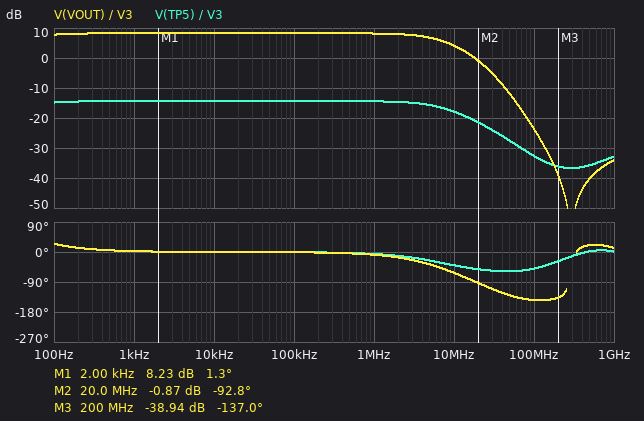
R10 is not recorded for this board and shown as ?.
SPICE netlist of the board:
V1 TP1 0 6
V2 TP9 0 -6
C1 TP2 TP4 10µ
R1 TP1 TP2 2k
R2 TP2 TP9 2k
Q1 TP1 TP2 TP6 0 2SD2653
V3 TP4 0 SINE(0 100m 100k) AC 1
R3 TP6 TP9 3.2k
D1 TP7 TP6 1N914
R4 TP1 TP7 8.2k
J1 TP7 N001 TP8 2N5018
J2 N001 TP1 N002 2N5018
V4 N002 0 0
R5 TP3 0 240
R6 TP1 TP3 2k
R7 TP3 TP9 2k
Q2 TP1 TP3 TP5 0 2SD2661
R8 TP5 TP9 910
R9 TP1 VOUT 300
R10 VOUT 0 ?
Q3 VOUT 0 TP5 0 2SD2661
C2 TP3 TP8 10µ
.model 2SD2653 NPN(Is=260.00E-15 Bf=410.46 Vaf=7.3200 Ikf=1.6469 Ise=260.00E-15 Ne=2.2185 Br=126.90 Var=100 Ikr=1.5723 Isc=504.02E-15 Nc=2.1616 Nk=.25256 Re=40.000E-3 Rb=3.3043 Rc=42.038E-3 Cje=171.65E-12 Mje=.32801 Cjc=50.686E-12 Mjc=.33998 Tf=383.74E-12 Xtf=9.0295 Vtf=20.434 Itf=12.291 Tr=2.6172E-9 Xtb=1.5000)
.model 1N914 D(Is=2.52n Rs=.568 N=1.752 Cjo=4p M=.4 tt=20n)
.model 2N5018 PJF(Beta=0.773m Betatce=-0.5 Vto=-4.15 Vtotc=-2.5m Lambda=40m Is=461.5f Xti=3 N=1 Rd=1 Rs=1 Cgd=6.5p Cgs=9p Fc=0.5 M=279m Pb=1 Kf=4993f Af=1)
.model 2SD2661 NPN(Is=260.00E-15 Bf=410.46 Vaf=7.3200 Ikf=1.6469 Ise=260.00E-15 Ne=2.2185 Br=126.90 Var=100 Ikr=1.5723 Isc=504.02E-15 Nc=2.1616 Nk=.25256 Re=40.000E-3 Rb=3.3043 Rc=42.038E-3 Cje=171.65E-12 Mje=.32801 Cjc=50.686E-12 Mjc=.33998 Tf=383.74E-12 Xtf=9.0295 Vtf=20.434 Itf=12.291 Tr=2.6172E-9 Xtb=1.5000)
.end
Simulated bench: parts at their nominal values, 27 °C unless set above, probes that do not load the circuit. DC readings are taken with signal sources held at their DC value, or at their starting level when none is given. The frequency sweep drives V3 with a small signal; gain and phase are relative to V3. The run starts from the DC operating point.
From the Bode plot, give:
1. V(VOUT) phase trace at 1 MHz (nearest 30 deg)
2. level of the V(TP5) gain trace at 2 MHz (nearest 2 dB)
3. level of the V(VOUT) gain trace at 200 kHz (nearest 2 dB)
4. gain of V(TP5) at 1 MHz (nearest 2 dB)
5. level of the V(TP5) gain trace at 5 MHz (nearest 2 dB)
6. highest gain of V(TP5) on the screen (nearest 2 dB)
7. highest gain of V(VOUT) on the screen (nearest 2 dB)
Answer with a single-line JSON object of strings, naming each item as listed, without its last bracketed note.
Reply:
{"V(VOUT) phase trace at 1 MHz": "0 deg", "level of the V(TP5) gain trace at 2 MHz": "-14 dB", "level of the V(VOUT) gain trace at 200 kHz": "8 dB", "gain of V(TP5) at 1 MHz": "-14 dB", "level of the V(TP5) gain trace at 5 MHz": "-16 dB", "highest gain of V(TP5) on the screen": "-14 dB", "highest gain of V(VOUT) on the screen": "8 dB"}
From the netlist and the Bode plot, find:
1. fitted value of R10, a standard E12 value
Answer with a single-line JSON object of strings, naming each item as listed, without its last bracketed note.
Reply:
{"fitted value of R10, a standard E12 value": "270 Ω"}
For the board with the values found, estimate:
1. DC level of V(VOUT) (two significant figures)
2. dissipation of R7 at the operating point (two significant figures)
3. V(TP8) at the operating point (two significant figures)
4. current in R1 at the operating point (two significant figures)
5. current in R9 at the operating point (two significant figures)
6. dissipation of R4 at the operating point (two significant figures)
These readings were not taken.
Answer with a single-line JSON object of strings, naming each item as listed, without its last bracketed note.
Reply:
{"DC level of V(VOUT)": "2.5 V", "dissipation of R7 at the operating point": "18 mW", "V(TP8) at the operating point": "14 mV", "current in R1 at the operating point": "3.0 mA", "current in R9 at the operating point": "12 mA", "dissipation of R4 at the operating point": "4.4 mW"}
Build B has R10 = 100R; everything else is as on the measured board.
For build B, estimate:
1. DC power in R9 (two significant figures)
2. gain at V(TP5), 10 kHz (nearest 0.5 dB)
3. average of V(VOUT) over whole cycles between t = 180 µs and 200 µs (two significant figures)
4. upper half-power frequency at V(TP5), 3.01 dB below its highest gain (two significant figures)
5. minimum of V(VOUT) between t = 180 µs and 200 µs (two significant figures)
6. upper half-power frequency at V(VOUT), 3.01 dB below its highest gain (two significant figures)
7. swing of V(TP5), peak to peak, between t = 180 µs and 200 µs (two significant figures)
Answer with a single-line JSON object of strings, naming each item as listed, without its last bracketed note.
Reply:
{"DC power in R9": "73 mW", "gain at V(TP5), 10 kHz": "-14.0 dB", "average of V(VOUT) over whole cycles between t = 180 µs and 200 µs": "1.3 V", "upper half-power frequency at V(TP5), 3.01 dB below its highest gain": "9.3 MHz", "minimum of V(VOUT) between t = 180 µs and 200 µs": "1.2 V", "upper half-power frequency at V(VOUT), 3.01 dB below its highest gain": "8.8 MHz", "swing of V(TP5), peak to peak, between t = 180 µs and 200 µs": "39 mV"}
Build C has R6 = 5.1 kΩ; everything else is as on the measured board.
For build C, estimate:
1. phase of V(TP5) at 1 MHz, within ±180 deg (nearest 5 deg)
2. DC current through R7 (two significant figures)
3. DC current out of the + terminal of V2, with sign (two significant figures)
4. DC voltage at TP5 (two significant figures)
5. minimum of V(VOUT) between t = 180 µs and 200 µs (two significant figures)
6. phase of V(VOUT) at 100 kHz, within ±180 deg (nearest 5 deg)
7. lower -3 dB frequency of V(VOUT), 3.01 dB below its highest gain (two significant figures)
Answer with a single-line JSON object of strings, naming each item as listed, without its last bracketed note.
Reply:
{"phase of V(TP5) at 1 MHz, within ±180 deg": "80 deg", "DC current through R7": "2.8 mA", "DC current out of the + terminal of V2, with sign": "-13 mA", "DC voltage at TP5": "-610 mV", "minimum of V(VOUT) between t = 180 µs and 200 µs": "2.0 V", "phase of V(VOUT) at 100 kHz, within ±180 deg": "90 deg", "lower -3 dB frequency of V(VOUT), 3.01 dB below its highest gain": "4.8 MHz"}
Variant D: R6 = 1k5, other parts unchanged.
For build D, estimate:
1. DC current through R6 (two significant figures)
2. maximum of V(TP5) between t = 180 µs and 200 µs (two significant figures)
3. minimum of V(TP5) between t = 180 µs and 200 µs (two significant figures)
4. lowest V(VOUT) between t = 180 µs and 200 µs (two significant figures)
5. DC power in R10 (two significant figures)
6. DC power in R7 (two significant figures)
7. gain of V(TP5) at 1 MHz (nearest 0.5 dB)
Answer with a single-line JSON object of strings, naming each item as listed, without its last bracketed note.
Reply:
{"DC current through R6": "3.9 mA", "maximum of V(TP5) between t = 180 µs and 200 µs": "-380 mV", "minimum of V(TP5) between t = 180 µs and 200 µs": "-450 mV", "lowest V(VOUT) between t = 180 µs and 200 µs": "2.8 V", "DC power in R10": "30 mW", "DC power in R7": "19 mW", "gain of V(TP5) at 1 MHz": "-9.5 dB"}
